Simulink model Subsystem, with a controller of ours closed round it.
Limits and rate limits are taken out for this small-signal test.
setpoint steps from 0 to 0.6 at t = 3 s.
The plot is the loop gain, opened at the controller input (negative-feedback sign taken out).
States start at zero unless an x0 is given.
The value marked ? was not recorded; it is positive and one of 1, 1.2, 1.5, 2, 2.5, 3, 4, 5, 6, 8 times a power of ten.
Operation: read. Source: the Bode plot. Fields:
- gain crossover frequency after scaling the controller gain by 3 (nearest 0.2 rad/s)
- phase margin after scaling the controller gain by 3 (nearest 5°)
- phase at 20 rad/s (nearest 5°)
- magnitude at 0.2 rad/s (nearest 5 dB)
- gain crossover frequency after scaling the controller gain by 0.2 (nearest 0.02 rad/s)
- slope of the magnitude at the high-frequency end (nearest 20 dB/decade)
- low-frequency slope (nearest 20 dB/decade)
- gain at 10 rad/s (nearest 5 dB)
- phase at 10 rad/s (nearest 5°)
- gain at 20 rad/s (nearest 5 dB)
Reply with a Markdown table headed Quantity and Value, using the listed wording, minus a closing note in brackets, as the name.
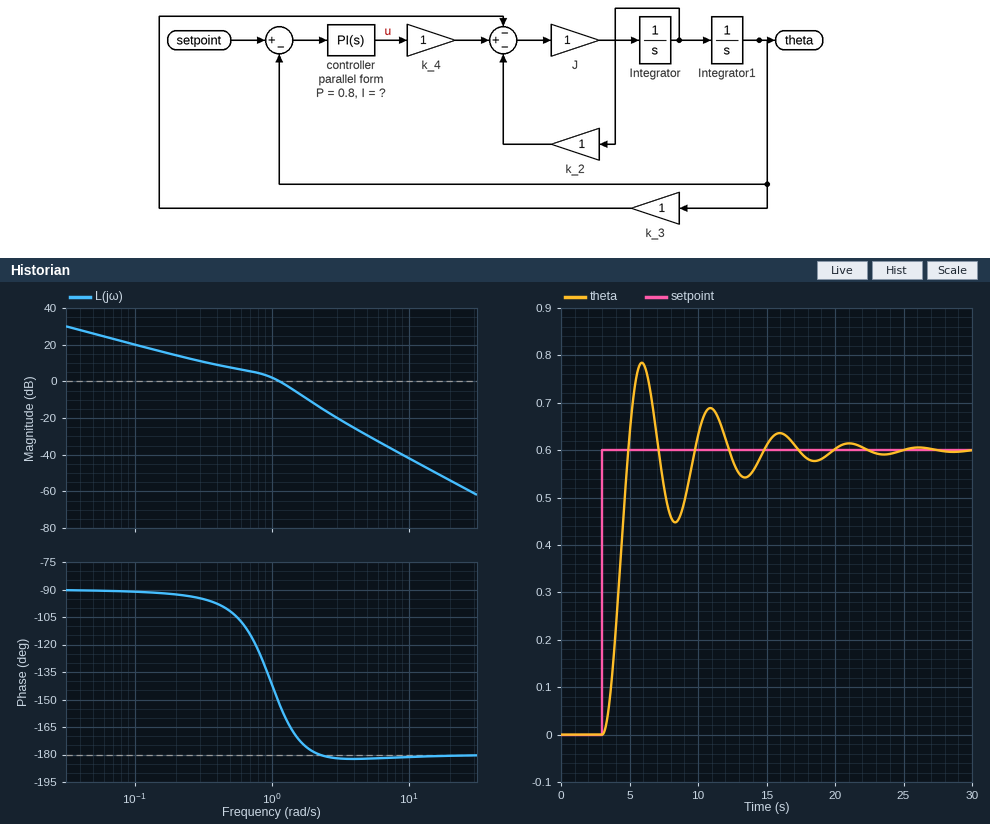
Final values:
| Quantity | Value |
|---|---|
| gain crossover frequency after scaling the controller gain by 3 | 1.8 rad/s |
| phase margin after scaling the controller gain by 3 | 5° |
| phase at 20 rad/s | -180° |
| magnitude at 0.2 rad/s | 15 dB |
| gain crossover frequency after scaling the controller gain by 0.2 | 0.20 rad/s |
| slope of the magnitude at the high-frequency end | -40 dB/decade |
| low-frequency slope | -20 dB/decade |
| gain at 10 rad/s | -40 dB |
| phase at 10 rad/s | -180° |
| gain at 20 rad/s | -55 dB |
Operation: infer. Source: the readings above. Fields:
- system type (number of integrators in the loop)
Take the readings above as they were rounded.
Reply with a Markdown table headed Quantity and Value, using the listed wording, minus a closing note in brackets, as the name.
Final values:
| Quantity | Value |
|---|---|
| system type | 1 |
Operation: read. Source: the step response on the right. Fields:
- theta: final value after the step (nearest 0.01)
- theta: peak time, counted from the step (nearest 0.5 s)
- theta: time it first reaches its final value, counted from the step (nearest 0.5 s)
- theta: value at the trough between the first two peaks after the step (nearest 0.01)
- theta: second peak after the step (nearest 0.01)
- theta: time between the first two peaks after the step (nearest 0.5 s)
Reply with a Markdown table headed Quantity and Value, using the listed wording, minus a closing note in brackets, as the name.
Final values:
| Quantity | Value |
|---|---|
| theta: final value after the step | 0.60 |
| theta: peak time, counted from the step | 3.0 s |
| theta: time it first reaches its final value, counted from the step | 2.0 s |
| theta: value at the trough between the first two peaks after the step | 0.45 |
| theta: second peak after the step | 0.69 |
| theta: time between the first two peaks after the step | 5.0 s |
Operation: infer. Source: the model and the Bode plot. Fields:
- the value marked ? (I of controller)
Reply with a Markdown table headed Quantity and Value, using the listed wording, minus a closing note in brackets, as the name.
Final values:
| Quantity | Value |
|---|---|
| the value marked ? | 1 |
